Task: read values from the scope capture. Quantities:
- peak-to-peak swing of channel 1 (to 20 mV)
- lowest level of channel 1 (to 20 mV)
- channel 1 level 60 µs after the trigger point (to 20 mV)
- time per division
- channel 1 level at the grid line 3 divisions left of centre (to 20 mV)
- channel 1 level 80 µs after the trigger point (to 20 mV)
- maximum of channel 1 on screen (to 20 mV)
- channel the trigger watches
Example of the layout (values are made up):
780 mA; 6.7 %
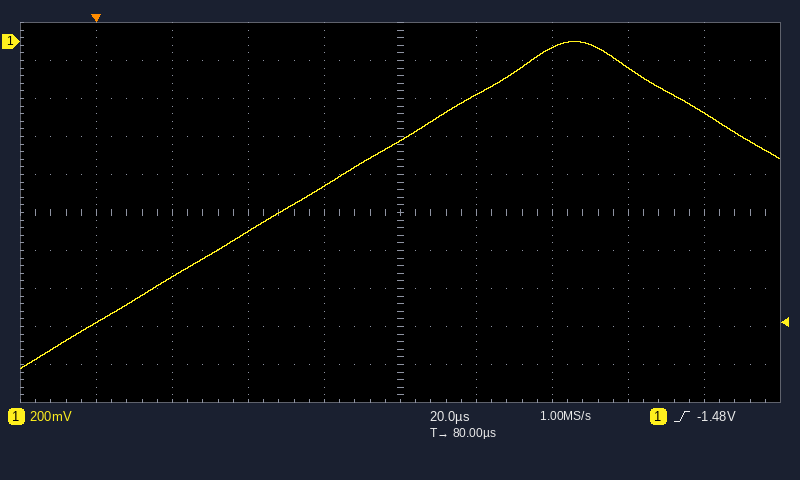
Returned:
1.72 V; -1.72 V; -760 mV; 20 µs; -1.24 V; -520 mV; 0 mV; channel 1
